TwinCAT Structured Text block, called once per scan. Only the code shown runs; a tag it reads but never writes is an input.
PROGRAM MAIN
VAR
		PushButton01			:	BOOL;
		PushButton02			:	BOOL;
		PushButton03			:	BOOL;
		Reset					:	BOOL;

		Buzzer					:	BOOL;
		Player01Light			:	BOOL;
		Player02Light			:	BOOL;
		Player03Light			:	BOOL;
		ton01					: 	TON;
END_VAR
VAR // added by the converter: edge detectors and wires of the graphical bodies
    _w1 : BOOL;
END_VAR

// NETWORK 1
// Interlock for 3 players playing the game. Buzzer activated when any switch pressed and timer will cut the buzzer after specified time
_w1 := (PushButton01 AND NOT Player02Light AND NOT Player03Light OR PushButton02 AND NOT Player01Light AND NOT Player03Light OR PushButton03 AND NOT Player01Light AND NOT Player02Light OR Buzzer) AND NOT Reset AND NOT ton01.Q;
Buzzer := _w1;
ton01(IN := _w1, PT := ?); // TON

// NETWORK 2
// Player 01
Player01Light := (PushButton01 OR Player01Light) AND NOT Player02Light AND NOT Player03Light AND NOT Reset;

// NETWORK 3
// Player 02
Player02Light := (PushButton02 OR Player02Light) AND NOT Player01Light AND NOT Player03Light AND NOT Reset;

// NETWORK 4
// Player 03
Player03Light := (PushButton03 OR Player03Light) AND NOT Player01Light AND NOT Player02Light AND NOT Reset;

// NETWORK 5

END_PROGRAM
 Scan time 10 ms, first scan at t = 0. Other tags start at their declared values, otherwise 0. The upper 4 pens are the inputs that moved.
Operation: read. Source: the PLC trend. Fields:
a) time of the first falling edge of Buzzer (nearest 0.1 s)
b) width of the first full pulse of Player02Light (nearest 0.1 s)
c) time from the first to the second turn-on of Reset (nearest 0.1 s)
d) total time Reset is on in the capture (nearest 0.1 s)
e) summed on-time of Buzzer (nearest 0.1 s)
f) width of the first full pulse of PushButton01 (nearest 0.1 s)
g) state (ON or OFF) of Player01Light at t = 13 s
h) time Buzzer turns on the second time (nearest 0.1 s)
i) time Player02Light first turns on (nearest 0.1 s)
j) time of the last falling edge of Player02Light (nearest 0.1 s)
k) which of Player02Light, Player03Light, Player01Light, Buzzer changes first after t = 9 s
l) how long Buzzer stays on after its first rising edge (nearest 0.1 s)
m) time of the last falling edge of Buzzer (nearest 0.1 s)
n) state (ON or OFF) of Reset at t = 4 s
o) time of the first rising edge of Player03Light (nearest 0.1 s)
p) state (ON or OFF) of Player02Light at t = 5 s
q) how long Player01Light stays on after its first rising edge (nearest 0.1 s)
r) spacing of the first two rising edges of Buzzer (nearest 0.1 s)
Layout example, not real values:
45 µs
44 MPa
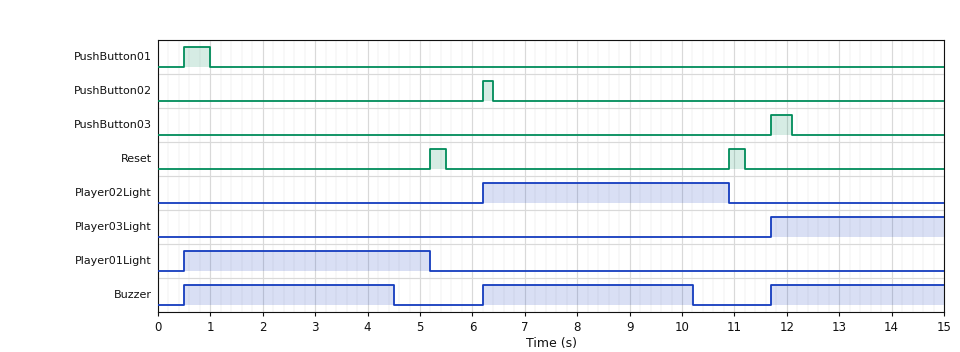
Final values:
4.5 s
4.7 s
5.7 s
0.6 s
11.3 s
0.5 s
OFF
6.2 s
6.2 s
10.9 s
Buzzer
4.0 s
10.2 s
OFF
11.7 s
OFF
4.7 s
5.7 s
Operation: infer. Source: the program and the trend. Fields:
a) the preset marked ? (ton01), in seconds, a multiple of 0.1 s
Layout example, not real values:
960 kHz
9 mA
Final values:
4.0 s
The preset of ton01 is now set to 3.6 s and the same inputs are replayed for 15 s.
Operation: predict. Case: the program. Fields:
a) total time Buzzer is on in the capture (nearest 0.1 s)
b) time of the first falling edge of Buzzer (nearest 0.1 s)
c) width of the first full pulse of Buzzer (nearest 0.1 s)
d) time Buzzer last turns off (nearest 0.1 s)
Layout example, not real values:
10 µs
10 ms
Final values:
10.5 s
4.1 s
3.6 s
9.8 s
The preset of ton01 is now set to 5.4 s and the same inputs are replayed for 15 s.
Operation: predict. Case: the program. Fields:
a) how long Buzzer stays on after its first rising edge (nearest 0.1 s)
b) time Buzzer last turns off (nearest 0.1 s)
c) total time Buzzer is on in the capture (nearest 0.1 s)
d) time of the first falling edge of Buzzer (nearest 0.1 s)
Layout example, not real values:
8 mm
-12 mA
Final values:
4.7 s
10.9 s
12.7 s
5.2 s
